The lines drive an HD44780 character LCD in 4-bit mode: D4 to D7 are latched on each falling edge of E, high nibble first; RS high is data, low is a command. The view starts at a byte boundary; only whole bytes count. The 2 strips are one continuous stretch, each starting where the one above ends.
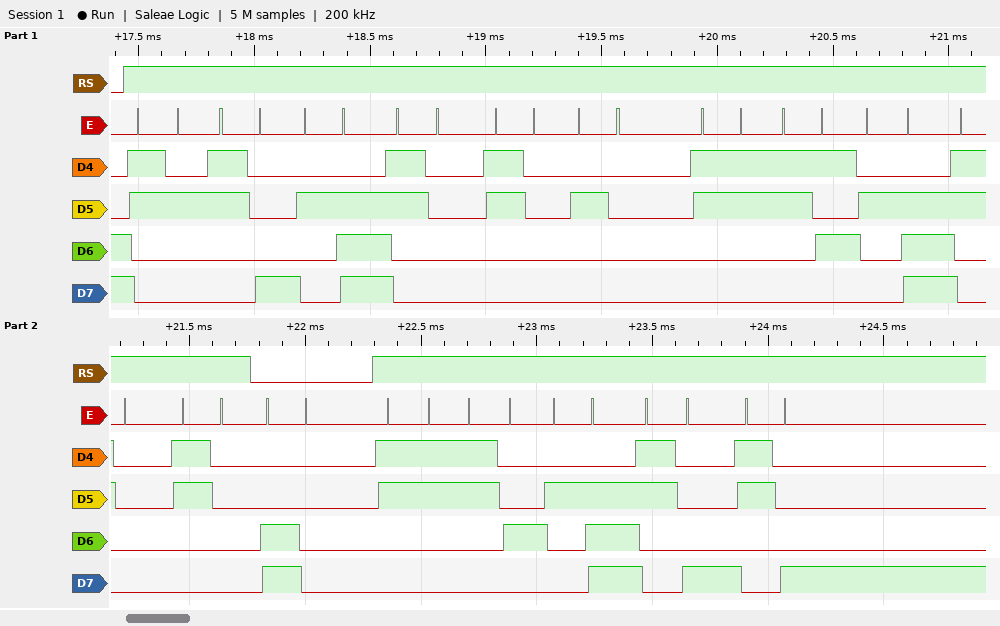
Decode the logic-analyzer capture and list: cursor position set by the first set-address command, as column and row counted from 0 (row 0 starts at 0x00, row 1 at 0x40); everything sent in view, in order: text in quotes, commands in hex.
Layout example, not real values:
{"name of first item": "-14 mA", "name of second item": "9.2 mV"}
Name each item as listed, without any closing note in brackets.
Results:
{"cursor position set by the first set-address command, as column and row counted from 0": "column 0, row 1", "everything sent in view, in order: text in quotes, commands in hex": "\"28.00 35.00\" 0xC0 \"34.88\""}
